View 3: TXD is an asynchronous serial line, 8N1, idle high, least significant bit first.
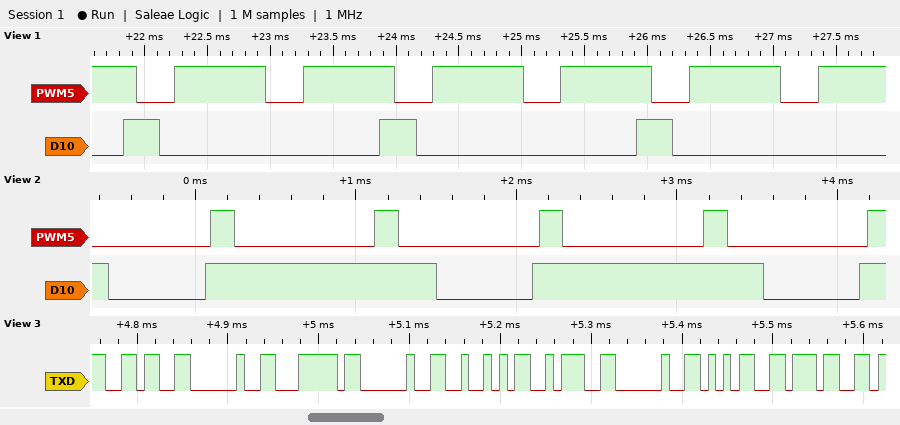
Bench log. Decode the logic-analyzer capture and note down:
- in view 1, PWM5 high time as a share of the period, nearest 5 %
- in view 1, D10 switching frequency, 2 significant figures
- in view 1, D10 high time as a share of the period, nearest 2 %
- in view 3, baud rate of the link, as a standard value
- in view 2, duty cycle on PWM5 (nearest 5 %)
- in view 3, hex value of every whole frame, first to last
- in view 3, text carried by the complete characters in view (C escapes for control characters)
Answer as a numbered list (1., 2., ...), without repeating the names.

1. 70 %
2. 490 Hz
3. 14 %
4. 115200 baud
5. 15 %
6. 36 20 7C 20 52 3A 20 35 37
7. "6 | R: 57"
